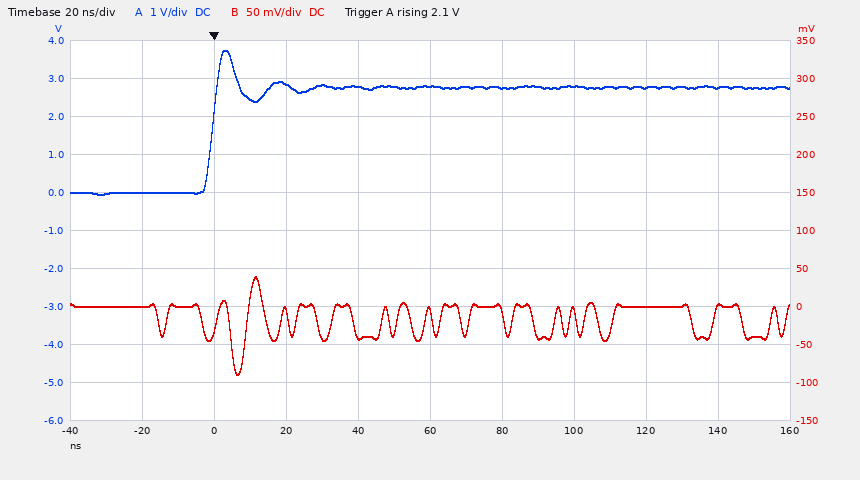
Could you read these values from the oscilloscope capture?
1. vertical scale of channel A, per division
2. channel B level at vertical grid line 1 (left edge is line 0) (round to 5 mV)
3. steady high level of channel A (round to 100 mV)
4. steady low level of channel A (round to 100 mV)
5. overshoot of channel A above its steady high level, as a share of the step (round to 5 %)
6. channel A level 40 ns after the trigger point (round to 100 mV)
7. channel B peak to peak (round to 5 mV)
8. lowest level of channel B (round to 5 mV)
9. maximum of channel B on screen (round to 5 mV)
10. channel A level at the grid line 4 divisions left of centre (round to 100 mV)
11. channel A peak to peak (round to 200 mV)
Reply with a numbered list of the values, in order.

1. 1 V
2. 0 mV
3. 2.8 V
4. 0.0 V
5. 35 %
6. 2.8 V
7. 130 mV
8. -90 mV
9. 40 mV
10. 0.0 V
11. 3.8 V
